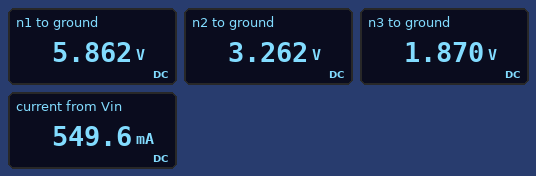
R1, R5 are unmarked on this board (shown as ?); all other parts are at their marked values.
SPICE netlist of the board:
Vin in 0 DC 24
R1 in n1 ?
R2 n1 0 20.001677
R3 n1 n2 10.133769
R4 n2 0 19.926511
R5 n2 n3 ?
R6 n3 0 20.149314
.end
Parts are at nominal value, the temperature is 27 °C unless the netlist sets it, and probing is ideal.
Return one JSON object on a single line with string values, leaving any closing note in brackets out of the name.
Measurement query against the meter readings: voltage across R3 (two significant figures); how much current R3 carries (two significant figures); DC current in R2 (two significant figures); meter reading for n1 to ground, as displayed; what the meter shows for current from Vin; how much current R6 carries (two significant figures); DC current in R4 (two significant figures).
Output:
{"voltage across R3": "2.6 V", "how much current R3 carries": "260 mA", "DC current in R2": "290 mA", "meter reading for n1 to ground, as displayed": "5.862 V", "what the meter shows for current from Vin": "549.6 mA", "how much current R6 carries": "93 mA", "DC current in R4": "160 mA"}
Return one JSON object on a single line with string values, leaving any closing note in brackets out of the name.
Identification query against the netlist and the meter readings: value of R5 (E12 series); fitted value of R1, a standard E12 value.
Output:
{"value of R5": "15 Ω", "fitted value of R1, a standard E12 value": "33 Ω"}
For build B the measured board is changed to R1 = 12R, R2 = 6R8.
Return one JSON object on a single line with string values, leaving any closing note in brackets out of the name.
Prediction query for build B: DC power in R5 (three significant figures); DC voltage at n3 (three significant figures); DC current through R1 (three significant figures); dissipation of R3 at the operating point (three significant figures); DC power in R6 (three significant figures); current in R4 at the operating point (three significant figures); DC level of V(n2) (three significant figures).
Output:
{"DC power in R5": "200 mW", "DC voltage at n3": "2.33 V", "DC current through R1": "1.39 A", "dissipation of R3 at the operating point": "1.03 W", "DC power in R6": "269 mW", "current in R4 at the operating point": "204 mA", "DC level of V(n2)": "4.06 V"}
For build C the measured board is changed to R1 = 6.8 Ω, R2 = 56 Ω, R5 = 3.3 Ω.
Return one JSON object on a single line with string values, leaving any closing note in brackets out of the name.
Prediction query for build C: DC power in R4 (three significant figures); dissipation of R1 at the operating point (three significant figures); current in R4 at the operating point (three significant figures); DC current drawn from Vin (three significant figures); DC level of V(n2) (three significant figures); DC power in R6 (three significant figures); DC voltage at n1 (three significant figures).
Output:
{"DC power in R4": "3.67 W", "dissipation of R1 at the operating point": "8.08 W", "current in R4 at the operating point": "429 mA", "DC current drawn from Vin": "1.09 A", "DC level of V(n2)": "8.55 V", "DC power in R6": "2.68 W", "DC voltage at n1": "16.6 V"}
